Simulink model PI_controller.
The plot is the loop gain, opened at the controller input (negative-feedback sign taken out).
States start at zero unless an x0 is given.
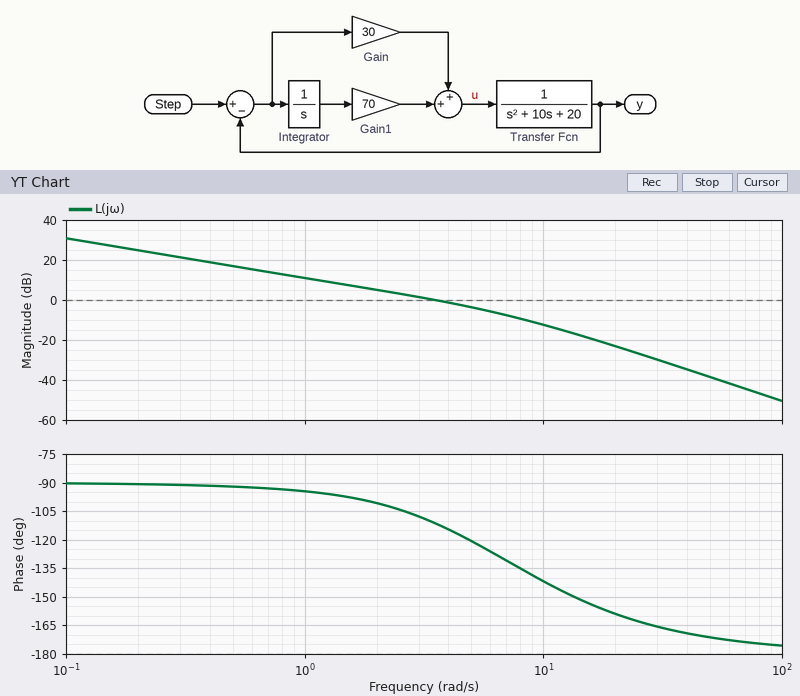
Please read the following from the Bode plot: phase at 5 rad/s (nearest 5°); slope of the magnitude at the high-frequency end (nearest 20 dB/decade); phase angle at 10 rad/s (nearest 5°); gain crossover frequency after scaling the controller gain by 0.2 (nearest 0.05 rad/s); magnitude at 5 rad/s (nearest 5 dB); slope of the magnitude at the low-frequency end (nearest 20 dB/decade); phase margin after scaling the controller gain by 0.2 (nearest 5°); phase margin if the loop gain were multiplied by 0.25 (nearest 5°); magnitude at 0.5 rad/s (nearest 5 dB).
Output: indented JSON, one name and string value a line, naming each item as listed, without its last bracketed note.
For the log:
{
  "phase at 5 rad/s": "-120°",
  "slope of the magnitude at the high-frequency end": "-40 dB/decade",
  "phase angle at 10 rad/s": "-140°",
  "gain crossover frequency after scaling the controller gain by 0.2": "0.70 rad/s",
  "magnitude at 5 rad/s": "-5 dB",
  "slope of the magnitude at the low-frequency end": "-20 dB/decade",
  "phase margin after scaling the controller gain by 0.2": "85°",
  "phase margin if the loop gain were multiplied by 0.25": "85°",
  "magnitude at 0.5 rad/s": "15 dB"
}
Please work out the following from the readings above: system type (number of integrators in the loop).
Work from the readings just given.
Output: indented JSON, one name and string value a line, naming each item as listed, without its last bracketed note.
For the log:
{
  "system type": "1"
}
